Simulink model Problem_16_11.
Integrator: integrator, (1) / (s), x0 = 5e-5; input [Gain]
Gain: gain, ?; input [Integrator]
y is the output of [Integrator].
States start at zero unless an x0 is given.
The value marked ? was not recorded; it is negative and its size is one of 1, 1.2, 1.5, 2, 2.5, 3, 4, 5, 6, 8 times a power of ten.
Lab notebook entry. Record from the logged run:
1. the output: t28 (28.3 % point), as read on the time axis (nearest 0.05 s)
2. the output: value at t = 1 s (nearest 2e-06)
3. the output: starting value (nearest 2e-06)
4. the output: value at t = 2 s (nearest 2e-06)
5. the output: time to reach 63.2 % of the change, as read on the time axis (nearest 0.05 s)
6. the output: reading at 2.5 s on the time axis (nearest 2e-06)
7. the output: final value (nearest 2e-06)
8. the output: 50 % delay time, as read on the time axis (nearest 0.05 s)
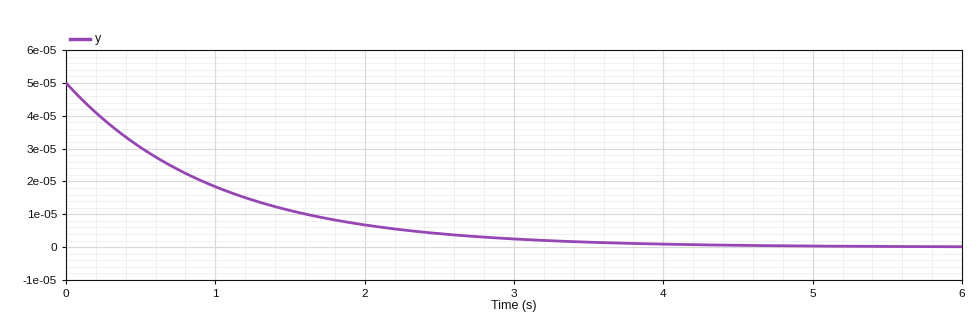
0.35 s
0.000018
0.000050
0.000006
1.00 s
0.000004
0.000000
0.70 s
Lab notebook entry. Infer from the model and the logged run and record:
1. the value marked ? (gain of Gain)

-1
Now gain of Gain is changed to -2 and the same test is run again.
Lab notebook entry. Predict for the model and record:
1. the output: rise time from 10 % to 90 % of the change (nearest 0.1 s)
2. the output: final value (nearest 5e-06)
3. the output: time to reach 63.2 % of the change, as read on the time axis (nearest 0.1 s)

1.1 s
0.000000
0.5 s
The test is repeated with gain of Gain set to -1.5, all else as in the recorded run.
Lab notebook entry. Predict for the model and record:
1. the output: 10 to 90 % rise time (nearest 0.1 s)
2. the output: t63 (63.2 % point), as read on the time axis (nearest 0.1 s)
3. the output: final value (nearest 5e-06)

1.5 s
0.7 s
0.000000
